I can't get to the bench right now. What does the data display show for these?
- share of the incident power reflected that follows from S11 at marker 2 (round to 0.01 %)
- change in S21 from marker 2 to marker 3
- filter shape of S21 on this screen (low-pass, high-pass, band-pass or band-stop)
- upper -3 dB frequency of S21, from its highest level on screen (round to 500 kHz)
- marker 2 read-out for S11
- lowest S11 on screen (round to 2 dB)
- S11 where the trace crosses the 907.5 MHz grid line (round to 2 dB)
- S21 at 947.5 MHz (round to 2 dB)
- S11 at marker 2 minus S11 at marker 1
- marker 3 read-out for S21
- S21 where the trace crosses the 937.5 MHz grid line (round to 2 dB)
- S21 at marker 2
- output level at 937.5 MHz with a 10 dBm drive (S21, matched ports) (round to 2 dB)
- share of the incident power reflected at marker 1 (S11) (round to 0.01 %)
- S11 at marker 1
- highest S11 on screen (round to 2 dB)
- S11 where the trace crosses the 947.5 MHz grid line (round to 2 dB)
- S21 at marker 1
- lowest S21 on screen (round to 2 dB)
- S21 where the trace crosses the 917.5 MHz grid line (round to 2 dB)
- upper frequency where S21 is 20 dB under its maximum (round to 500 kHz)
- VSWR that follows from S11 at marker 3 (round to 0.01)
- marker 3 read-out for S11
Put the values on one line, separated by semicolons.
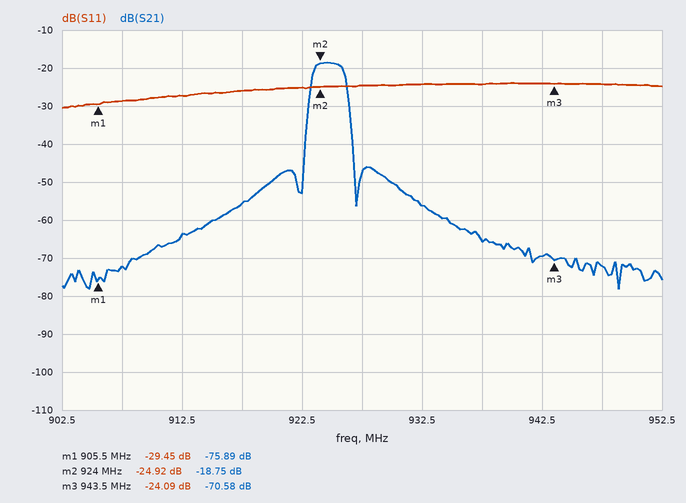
0.32 %; -51.83 dB; band-pass; 926.0 MHz; -24.92 dB; -30 dB; -28 dB; -72 dB; 4.53 dB; -70.58 dB; -66 dB; -18.75 dB; -56 dBm; 0.11 %; -29.45 dB; -24 dB; -24 dB; -75.89 dB; -78 dB; -56 dB; 926.5 MHz; 1.13; -24.09 dB
